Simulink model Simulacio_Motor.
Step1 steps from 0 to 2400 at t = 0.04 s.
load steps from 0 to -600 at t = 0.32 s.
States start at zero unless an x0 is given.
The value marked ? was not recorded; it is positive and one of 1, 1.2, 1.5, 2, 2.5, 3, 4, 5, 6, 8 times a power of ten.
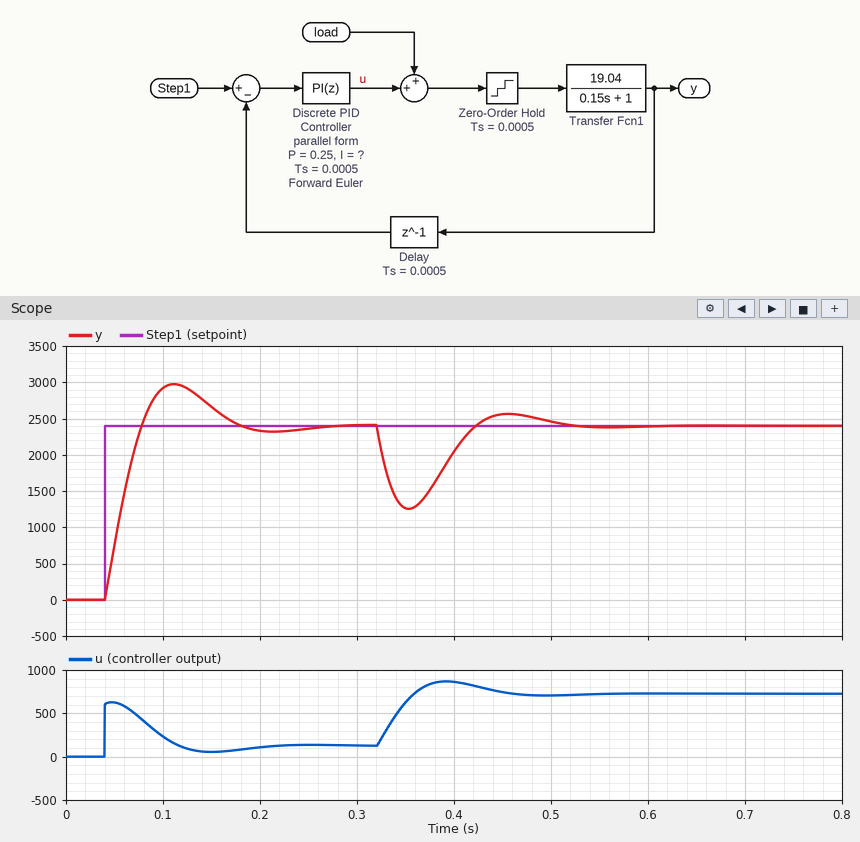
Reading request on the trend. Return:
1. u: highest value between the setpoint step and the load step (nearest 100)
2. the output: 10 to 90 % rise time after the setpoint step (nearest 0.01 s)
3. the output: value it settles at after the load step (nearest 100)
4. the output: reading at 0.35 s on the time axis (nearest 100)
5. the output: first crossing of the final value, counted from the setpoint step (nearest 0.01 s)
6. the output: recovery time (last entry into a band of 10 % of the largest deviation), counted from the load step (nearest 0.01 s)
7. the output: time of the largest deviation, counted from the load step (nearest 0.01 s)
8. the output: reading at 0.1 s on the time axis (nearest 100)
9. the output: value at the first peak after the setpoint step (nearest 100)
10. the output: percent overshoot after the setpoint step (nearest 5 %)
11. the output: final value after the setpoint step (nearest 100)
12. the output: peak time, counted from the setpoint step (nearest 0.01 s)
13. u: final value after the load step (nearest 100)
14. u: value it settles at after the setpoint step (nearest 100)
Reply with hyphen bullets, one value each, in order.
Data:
- 600
- 0.03 s
- 2400
- 1300
- 0.04 s
- 0.16 s
- 0.03 s
- 2900
- 3000
- 25 %
- 2400
- 0.07 s
- 700
- 100
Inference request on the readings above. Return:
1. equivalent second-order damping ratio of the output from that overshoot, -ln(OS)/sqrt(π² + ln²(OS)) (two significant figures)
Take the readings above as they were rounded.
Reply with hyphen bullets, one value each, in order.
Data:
- 0.40
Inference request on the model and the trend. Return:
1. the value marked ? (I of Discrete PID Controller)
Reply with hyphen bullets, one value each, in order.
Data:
- 10
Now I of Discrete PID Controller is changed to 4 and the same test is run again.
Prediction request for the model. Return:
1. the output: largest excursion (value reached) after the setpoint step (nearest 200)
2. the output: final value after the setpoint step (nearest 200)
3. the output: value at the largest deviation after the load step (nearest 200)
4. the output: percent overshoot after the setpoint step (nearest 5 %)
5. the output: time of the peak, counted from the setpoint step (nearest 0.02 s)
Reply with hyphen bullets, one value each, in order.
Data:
- 2600
- 2400
- 1000
- 10 %
- 0.10 s
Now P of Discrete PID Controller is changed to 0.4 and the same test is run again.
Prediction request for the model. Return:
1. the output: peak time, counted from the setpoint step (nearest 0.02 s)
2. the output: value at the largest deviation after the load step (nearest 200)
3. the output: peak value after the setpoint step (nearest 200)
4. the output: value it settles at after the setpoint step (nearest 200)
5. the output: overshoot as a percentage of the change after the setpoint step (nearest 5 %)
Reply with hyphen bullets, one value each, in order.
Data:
- 0.06 s
- 1400
- 2800
- 2400
- 15 %
